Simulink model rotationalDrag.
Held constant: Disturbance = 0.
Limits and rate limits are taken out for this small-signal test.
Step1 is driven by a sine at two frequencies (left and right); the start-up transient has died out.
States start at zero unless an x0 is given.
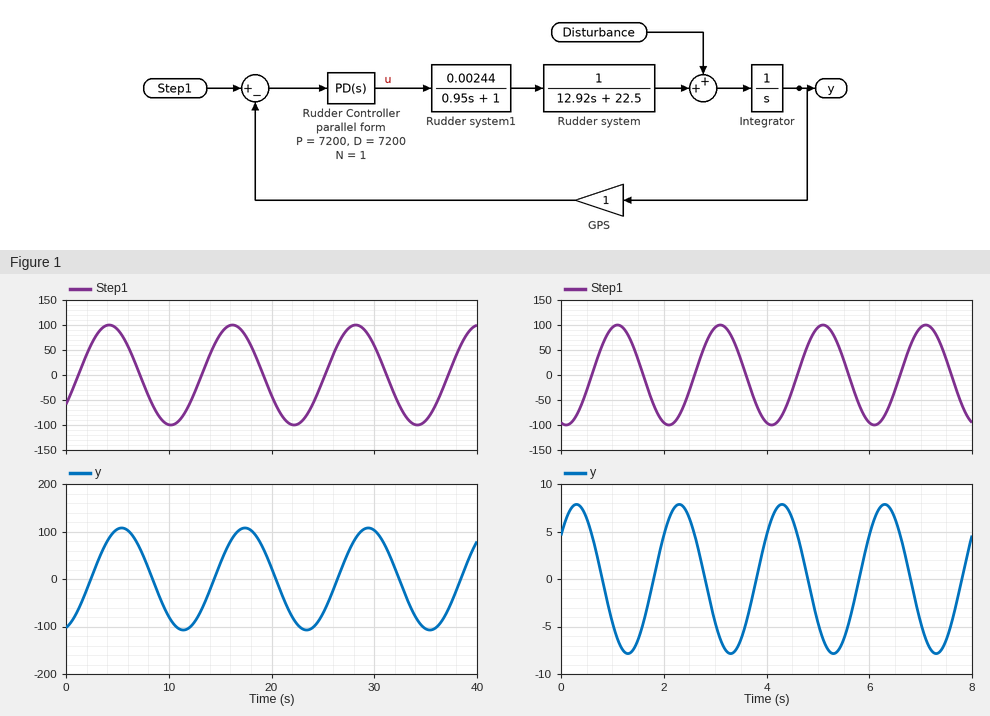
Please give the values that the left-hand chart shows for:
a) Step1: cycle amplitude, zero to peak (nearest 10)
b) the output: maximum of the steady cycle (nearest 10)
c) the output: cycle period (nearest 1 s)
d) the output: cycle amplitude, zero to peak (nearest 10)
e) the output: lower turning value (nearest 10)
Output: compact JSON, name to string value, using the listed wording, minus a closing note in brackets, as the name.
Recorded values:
{"Step1: cycle amplitude, zero to peak": "100", "the output: maximum of the steady cycle": "110", "the output: cycle period": "12 s", "the output: cycle amplitude, zero to peak": "110", "the output: lower turning value": "-110"}
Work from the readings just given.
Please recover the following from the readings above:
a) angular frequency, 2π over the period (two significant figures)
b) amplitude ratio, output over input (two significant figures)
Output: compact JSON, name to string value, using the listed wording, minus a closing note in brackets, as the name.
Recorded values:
{"angular frequency, 2π over the period": "0.52 rad/s", "amplitude ratio, output over input": "1.1"}
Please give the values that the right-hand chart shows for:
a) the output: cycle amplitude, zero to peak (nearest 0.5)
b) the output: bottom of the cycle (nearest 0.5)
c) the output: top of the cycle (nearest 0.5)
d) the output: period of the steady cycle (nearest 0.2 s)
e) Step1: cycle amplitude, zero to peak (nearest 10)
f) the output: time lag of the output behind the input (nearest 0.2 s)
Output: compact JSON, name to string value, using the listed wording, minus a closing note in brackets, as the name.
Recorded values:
{"the output: cycle amplitude, zero to peak": "8.0", "the output: bottom of the cycle": "-8.0", "the output: top of the cycle": "8.0", "the output: period of the steady cycle": "2.0 s", "Step1: cycle amplitude, zero to peak": "100", "the output: time lag of the output behind the input": "1.2 s"}
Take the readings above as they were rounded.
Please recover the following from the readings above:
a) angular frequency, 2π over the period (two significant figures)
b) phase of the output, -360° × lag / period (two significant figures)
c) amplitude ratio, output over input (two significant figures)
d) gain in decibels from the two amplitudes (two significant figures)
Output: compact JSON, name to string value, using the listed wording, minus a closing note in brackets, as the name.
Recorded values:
{"angular frequency, 2π over the period": "3.1 rad/s", "phase of the output, -360° × lag / period": "-220°", "amplitude ratio, output over input": "0.080", "gain in decibels from the two amplitudes": "-22 dB"}
